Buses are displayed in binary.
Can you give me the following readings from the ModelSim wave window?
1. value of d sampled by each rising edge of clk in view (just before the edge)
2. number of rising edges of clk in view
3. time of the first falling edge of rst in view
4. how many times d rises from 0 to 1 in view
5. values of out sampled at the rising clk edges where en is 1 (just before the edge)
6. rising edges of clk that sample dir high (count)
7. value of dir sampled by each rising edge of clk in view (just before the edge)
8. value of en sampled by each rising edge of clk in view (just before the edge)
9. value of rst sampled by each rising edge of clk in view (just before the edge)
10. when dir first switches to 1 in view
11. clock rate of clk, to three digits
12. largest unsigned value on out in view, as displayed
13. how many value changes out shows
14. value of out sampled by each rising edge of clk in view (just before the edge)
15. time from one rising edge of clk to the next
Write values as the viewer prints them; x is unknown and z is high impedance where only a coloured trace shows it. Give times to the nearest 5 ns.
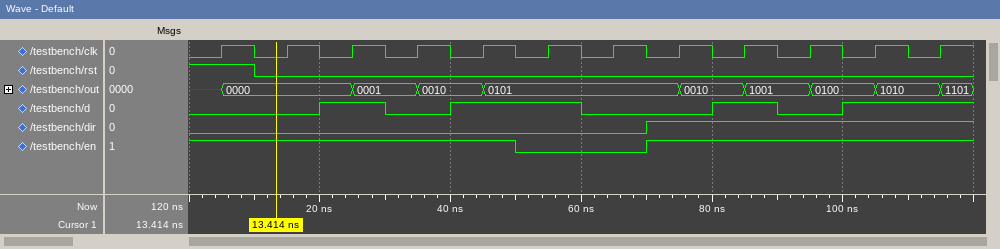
0 0 1 0 1 1 0 0 1 0 1 1
12
10 ns
4
x, 0000, 0000, 0001, 0010, 0101, 0010, 1001, 0100, 1010
5
0 0 0 0 0 0 0 1 1 1 1 1
1 1 1 1 1 0 0 1 1 1 1 1
1 0 0 0 0 0 0 0 0 0 0 0
70 ns
100 MHz
1101
9
x, 0000, 0000, 0001, 0010, 0101, 0101, 0101, 0010, 1001, 0100, 1010
10 ns
